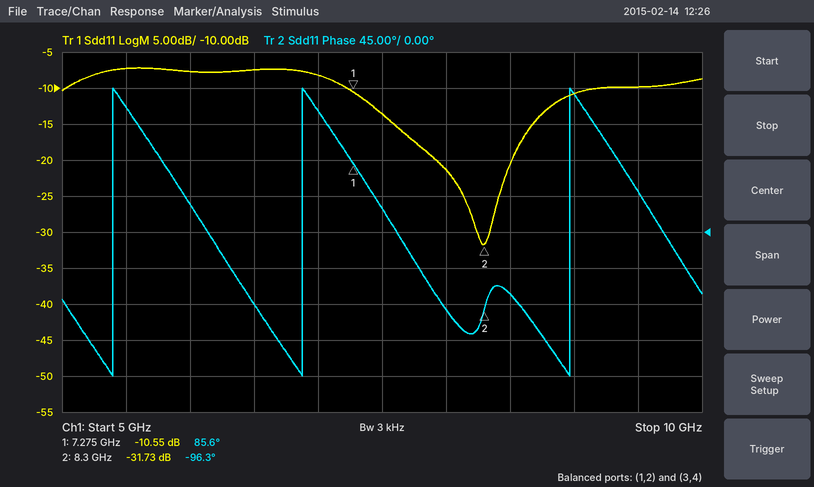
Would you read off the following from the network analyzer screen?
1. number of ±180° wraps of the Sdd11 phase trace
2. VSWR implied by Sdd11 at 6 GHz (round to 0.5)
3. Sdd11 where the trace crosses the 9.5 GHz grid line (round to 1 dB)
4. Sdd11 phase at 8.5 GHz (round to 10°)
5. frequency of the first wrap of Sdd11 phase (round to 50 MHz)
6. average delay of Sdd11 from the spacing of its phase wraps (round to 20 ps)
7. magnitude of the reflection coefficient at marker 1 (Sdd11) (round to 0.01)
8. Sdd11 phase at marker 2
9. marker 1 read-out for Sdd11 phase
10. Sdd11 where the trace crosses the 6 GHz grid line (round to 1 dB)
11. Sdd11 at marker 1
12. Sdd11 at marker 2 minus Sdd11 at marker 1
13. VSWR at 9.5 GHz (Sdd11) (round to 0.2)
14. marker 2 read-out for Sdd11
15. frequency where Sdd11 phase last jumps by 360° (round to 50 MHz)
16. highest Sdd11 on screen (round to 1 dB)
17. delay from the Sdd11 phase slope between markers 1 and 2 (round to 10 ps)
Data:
3
2.5
-10 dB
-80°
5.40 GHz
560 ps
0.30
-96.3°
85.6°
-8 dB
-10.55 dB
-21.18 dB
2.0
-31.73 dB
8.95 GHz
-7 dB
490 ps
